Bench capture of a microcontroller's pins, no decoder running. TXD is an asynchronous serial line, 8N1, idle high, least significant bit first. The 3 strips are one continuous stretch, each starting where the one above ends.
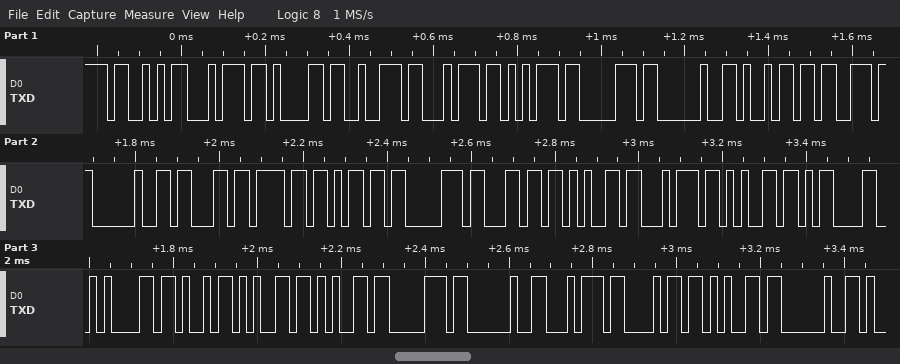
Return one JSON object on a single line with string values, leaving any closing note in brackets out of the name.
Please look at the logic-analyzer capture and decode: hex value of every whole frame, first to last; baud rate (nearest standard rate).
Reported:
{"hex value of every whole frame, first to last": "53 74 61 72 74 75 70 20 69 73 20 63 6F 6D 70 6C 65 74 65 0D 0A 4B 65 65 70 20 74 68 65 20", "baud rate": "57600 baud"}
